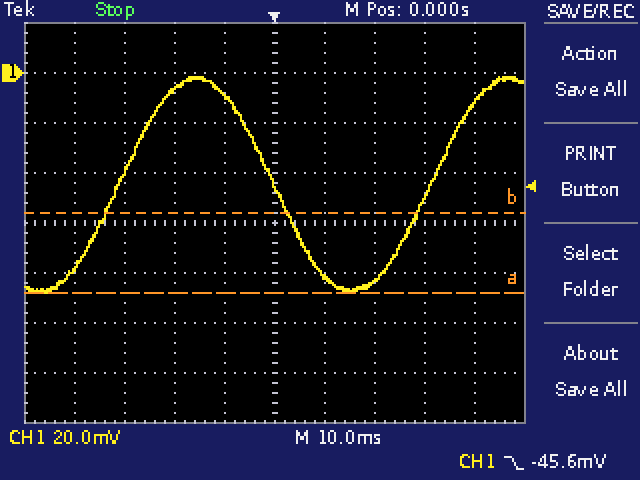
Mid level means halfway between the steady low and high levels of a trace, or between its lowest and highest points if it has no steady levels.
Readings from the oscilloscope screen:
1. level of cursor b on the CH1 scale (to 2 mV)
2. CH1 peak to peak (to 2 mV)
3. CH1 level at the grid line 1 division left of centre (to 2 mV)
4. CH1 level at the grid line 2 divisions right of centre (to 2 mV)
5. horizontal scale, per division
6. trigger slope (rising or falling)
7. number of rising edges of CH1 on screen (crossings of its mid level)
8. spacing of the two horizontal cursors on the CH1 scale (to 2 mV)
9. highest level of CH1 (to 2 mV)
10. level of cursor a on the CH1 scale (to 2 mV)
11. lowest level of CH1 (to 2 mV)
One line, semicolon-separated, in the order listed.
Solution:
-56 mV; 86 mV; -8 mV; -84 mV; 10 ms; falling; 2; 32 mV; -2 mV; -88 mV; -88 mV
